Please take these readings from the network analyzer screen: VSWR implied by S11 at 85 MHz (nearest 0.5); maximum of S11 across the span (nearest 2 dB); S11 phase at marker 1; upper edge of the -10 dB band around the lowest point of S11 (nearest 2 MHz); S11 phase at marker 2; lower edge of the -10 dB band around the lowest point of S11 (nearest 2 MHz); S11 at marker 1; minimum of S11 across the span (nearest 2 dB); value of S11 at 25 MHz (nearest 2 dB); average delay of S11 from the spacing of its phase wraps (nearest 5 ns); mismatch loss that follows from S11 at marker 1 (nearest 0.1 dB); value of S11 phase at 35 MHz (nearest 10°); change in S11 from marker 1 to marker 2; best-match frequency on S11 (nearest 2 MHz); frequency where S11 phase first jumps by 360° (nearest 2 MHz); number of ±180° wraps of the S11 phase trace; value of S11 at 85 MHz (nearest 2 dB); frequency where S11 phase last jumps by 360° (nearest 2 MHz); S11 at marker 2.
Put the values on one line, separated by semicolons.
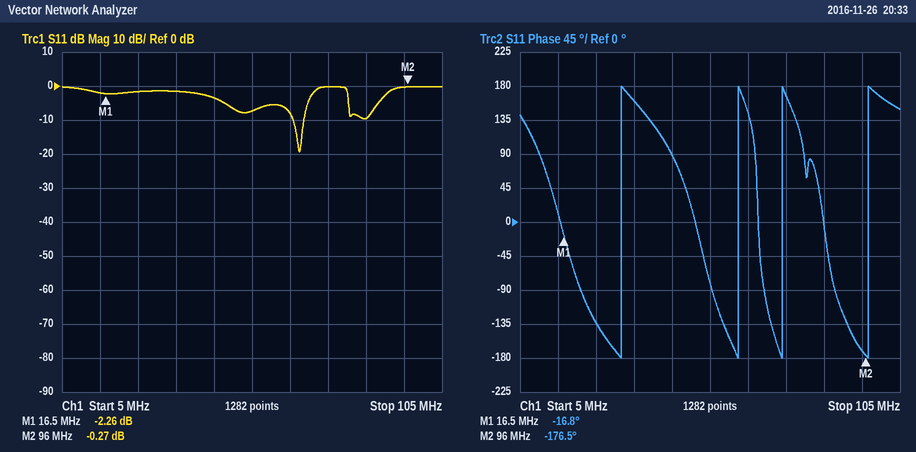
2.0; 0 dB; -16.8°; 68 MHz; -176.5°; 66 MHz; -2.26 dB; -20 dB; -2 dB; 45 ns; 3.9 dB; 160°; 1.99 dB; 68 MHz; 32 MHz; 4; -10 dB; 96 MHz; -0.27 dB
